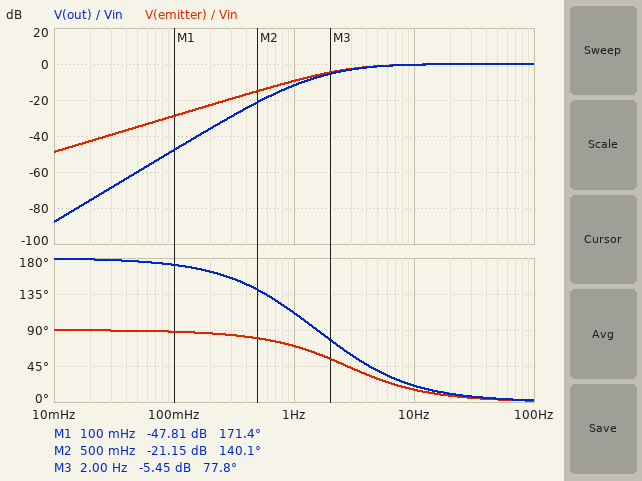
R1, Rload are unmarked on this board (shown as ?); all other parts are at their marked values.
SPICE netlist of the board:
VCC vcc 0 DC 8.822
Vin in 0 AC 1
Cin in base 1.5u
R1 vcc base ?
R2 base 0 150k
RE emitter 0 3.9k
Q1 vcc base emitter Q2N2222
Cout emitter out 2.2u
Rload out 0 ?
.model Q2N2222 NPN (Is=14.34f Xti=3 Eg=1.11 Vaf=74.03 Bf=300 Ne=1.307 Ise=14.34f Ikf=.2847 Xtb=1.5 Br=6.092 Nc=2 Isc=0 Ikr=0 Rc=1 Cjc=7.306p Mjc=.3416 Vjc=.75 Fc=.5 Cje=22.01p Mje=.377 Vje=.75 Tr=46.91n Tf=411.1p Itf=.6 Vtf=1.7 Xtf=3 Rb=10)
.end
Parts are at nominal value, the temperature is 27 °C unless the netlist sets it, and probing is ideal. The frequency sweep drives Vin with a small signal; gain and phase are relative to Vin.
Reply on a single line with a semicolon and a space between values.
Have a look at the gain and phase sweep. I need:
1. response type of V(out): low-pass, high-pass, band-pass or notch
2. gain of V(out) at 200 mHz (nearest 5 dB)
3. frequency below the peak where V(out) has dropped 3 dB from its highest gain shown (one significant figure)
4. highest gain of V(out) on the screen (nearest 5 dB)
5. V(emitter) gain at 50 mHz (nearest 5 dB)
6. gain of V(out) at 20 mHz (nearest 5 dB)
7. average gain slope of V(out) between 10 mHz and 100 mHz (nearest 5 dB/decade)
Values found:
high-pass; -35 dB; 3 Hz; 0 dB; -35 dB; -75 dB; 40 dB/decade
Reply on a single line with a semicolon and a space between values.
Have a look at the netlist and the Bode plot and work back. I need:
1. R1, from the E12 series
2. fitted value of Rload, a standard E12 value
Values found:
56 kΩ; 82 kΩ
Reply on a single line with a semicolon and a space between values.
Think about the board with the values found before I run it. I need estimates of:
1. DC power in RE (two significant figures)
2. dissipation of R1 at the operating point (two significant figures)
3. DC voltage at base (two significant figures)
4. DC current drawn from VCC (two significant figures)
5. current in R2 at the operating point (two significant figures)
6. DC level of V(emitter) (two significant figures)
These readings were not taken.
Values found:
7.6 mW; 130 µW; 6.1 V; 1.4 mA; 41 µA; 5.4 V
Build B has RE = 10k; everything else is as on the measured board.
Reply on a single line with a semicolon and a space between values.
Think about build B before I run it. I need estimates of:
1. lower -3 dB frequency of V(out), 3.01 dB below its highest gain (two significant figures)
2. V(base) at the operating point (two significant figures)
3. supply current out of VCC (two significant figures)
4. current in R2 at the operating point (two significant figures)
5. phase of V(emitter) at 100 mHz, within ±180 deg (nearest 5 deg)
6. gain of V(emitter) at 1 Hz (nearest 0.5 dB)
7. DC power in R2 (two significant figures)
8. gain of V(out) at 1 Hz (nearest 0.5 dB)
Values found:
2.9 Hz; 6.3 V; 610 µA; 42 µA; 90 deg; -9.0 dB; 260 µW; -11.5 dB
